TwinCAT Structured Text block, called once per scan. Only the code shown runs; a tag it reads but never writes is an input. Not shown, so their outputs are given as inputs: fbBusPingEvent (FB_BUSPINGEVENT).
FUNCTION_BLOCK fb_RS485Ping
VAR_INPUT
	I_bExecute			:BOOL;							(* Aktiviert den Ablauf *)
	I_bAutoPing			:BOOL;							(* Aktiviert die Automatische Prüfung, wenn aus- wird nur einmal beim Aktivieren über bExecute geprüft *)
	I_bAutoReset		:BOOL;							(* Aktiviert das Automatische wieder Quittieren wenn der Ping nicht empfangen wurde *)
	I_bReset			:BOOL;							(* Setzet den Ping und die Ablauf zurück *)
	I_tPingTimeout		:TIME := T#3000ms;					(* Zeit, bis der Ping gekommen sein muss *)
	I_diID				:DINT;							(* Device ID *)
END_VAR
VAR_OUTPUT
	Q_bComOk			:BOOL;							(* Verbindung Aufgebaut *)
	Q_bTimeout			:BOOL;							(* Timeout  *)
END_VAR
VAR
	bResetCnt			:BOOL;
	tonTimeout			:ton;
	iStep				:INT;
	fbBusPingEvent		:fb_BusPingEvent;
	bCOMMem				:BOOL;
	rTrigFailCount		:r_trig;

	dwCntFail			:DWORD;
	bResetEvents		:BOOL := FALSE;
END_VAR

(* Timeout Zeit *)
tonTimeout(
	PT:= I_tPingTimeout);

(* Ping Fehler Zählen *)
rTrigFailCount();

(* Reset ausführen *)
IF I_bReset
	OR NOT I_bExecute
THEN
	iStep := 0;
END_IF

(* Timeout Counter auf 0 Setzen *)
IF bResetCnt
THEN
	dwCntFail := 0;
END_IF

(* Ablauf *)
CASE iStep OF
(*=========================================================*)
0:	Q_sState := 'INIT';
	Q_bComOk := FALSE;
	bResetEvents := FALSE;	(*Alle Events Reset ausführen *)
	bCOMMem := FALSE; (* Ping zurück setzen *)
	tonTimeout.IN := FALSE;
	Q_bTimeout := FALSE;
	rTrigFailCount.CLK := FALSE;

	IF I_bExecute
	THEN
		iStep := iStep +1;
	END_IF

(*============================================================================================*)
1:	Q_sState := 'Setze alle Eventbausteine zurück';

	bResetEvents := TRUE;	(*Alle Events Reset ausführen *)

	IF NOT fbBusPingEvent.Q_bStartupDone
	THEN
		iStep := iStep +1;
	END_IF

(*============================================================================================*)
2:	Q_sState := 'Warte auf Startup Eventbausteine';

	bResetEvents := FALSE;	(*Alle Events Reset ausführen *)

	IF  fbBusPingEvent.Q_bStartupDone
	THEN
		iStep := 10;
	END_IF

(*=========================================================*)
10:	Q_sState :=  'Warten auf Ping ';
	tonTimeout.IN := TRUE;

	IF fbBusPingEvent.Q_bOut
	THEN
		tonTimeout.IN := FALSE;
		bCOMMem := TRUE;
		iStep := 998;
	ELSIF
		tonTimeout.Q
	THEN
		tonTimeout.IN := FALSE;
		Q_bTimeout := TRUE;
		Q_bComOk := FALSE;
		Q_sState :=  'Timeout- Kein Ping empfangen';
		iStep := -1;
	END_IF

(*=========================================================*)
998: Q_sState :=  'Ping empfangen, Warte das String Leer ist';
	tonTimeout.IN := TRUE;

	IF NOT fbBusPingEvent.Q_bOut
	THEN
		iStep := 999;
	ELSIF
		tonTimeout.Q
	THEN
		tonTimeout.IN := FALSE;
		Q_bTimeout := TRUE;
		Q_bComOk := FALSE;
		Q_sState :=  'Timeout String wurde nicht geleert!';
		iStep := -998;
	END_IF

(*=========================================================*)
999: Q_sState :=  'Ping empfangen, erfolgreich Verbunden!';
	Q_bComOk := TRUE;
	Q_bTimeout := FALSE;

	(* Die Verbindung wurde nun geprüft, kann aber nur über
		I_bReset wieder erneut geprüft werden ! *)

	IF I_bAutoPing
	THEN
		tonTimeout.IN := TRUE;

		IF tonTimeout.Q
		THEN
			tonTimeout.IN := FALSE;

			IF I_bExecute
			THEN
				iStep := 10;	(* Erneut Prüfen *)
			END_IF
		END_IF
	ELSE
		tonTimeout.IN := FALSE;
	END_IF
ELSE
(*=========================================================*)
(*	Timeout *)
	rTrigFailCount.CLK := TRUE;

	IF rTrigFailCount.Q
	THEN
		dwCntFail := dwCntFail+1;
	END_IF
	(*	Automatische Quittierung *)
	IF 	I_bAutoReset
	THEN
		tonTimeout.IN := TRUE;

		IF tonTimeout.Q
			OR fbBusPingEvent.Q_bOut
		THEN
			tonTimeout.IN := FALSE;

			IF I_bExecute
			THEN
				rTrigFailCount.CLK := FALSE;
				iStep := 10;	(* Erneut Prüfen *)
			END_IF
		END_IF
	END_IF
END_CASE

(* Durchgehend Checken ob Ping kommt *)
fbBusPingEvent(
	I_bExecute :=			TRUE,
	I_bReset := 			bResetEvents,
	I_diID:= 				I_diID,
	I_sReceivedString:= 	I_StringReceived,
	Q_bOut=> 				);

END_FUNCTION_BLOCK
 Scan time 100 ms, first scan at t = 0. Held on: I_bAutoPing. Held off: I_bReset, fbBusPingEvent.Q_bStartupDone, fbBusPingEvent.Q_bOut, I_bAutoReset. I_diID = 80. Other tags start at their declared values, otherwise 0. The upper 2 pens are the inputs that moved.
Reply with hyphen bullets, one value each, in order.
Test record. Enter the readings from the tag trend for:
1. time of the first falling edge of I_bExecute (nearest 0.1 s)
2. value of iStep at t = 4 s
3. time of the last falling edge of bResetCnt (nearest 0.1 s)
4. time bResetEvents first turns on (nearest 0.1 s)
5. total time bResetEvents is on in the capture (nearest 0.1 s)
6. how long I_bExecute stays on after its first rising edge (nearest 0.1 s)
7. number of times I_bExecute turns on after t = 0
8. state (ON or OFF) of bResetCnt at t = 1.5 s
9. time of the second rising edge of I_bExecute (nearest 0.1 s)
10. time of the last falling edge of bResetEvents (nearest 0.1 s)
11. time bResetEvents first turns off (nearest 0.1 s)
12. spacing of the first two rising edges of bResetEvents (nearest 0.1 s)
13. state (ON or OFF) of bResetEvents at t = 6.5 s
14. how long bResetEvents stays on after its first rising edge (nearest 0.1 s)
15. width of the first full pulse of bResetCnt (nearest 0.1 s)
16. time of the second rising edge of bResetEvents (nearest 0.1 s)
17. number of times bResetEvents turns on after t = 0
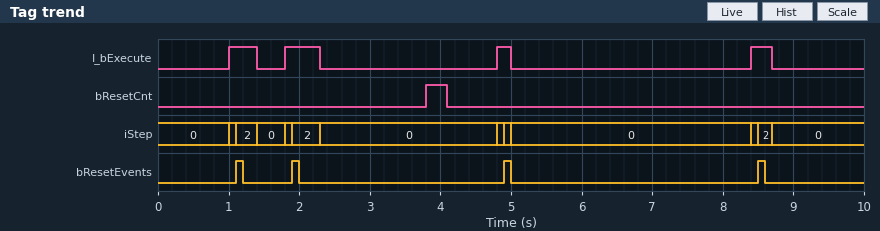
- 1.4 s
- 0
- 4.1 s
- 1.1 s
- 0.4 s
- 0.4 s
- 4
- OFF
- 1.8 s
- 8.6 s
- 1.2 s
- 0.8 s
- OFF
- 0.1 s
- 0.3 s
- 1.9 s
- 4
